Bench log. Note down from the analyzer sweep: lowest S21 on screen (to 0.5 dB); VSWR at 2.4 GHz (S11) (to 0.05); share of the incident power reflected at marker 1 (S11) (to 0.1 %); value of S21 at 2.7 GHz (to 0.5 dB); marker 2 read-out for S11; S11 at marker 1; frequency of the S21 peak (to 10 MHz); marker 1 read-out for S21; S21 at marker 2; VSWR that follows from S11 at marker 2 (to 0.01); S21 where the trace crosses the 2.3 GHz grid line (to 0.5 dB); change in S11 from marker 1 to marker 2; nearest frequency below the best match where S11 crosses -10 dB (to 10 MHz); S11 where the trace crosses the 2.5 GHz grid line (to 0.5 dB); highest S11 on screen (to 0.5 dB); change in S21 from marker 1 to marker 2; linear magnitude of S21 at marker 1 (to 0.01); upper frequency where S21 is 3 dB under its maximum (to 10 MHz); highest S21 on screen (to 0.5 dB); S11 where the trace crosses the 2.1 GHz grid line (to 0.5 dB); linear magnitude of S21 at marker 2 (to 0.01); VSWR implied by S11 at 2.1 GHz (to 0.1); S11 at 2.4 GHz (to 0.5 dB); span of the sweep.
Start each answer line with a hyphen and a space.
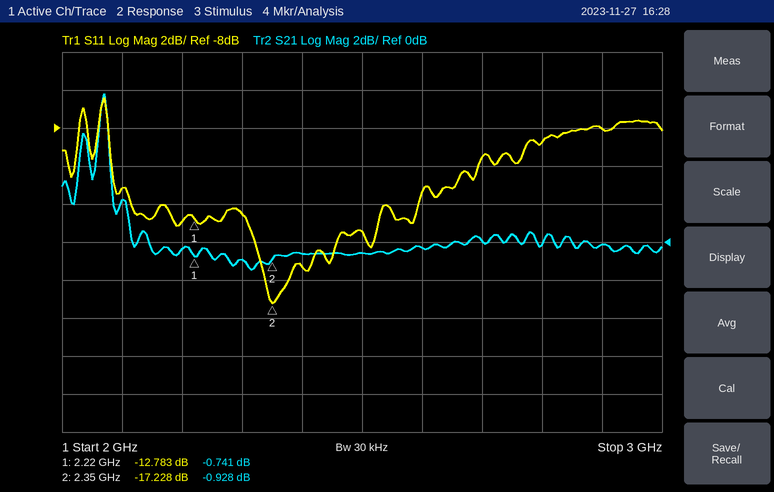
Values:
- -1.5 dB
- 1.40
- 5.3 %
- 0.0 dB
- -17.228 dB
- -12.783 dB
- 2.07 GHz
- -0.741 dB
- -0.928 dB
- 1.32
- -1.0 dB
- -4.445 dB
- 2.08 GHz
- -13.5 dB
- -6.5 dB
- -0.187 dB
- 0.92
- 2.08 GHz
- 8.0 dB
- -11.0 dB
- 0.90
- 1.8
- -15.5 dB
- 1 GHz
